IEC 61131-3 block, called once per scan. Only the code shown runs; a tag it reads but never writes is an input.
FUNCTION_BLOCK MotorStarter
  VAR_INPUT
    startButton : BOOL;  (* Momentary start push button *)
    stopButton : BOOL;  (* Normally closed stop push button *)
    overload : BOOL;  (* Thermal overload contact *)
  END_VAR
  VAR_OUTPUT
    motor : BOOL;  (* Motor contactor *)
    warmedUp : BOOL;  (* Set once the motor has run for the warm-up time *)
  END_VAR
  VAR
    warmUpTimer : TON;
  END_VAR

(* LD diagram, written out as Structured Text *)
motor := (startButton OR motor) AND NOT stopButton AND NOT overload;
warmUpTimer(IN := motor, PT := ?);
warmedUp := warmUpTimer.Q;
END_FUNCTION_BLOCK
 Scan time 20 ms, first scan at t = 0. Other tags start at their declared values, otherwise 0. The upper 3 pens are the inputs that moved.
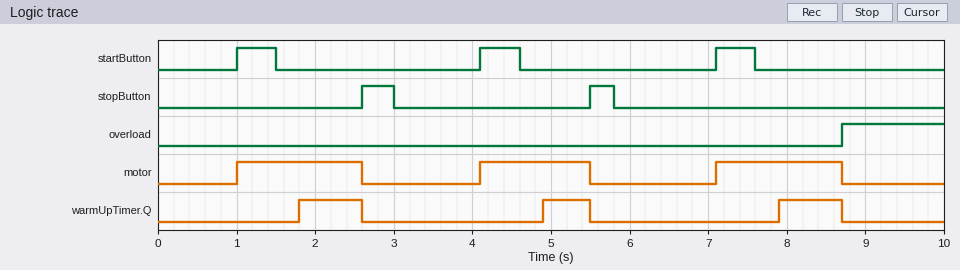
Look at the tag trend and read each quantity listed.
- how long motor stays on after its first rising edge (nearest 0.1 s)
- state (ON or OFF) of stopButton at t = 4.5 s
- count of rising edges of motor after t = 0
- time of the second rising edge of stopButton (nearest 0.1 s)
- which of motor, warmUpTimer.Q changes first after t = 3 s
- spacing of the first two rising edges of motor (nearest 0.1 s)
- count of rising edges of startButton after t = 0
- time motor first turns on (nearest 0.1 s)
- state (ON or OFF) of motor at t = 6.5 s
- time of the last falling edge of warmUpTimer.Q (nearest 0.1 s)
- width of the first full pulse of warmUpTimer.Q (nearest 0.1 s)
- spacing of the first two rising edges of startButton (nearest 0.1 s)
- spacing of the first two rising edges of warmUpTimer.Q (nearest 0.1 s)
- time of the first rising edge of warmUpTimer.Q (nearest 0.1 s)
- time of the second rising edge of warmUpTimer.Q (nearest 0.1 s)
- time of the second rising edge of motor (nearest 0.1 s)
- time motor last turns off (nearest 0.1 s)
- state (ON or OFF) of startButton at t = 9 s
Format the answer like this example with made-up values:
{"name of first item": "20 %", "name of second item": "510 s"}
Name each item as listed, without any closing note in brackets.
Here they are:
{"how long motor stays on after its first rising edge": "1.6 s", "state (ON or OFF) of stopButton at t = 4.5 s": "OFF", "count of rising edges of motor after t = 0": "3", "time of the second rising edge of stopButton": "5.5 s", "which of motor, warmUpTimer.Q changes first after t = 3 s": "motor", "spacing of the first two rising edges of motor": "3.1 s", "count of rising edges of startButton after t = 0": "3", "time motor first turns on": "1.0 s", "state (ON or OFF) of motor at t = 6.5 s": "OFF", "time of the last falling edge of warmUpTimer.Q": "8.7 s", "width of the first full pulse of warmUpTimer.Q": "0.8 s", "spacing of the first two rising edges of startButton": "3.1 s", "spacing of the first two rising edges of warmUpTimer.Q": "3.1 s", "time of the first rising edge of warmUpTimer.Q": "1.8 s", "time of the second rising edge of warmUpTimer.Q": "4.9 s", "time of the second rising edge of motor": "4.1 s", "time motor last turns off": "8.7 s", "state (ON or OFF) of startButton at t = 9 s": "OFF"}
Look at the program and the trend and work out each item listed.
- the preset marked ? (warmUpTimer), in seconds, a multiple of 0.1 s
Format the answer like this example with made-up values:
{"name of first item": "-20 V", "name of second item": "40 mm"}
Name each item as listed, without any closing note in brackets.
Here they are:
{"the preset marked ? (warmUpTimer), in seconds, a multiple of 0.1 s": "0.8 s"}
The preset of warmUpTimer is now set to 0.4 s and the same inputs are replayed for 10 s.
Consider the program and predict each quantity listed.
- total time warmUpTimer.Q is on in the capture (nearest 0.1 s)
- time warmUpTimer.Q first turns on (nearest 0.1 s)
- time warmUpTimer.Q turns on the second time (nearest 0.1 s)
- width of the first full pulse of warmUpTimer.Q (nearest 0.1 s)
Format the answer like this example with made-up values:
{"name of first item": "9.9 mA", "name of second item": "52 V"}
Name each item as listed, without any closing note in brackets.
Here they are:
{"total time warmUpTimer.Q is on in the capture": "3.4 s", "time warmUpTimer.Q first turns on": "1.4 s", "time warmUpTimer.Q turns on the second time": "4.5 s", "width of the first full pulse of warmUpTimer.Q": "1.2 s"}
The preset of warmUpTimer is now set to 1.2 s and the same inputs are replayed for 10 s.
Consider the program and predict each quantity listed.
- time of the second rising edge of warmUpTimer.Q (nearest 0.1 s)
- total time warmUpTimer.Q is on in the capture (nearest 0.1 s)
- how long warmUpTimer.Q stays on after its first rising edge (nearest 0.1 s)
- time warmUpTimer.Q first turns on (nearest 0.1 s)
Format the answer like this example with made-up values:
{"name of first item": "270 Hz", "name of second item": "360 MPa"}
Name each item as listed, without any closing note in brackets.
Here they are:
{"time of the second rising edge of warmUpTimer.Q": "5.3 s", "total time warmUpTimer.Q is on in the capture": "1.0 s", "how long warmUpTimer.Q stays on after its first rising edge": "0.4 s", "time warmUpTimer.Q first turns on": "2.2 s"}
